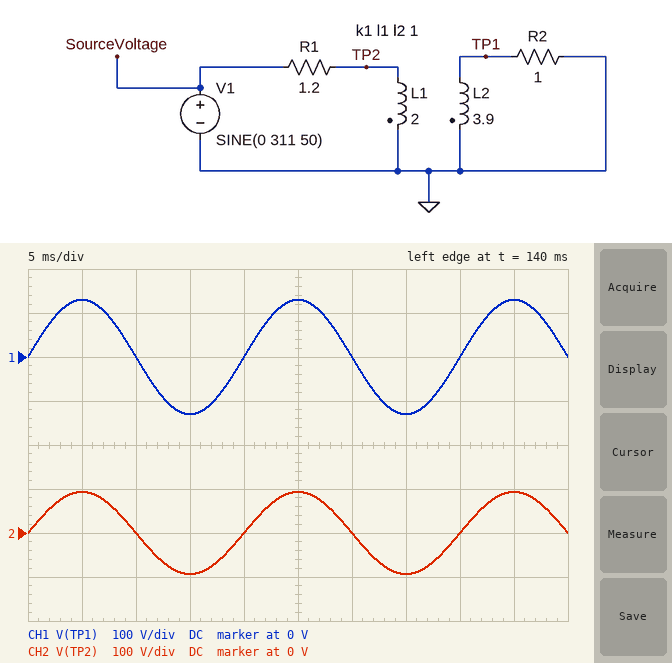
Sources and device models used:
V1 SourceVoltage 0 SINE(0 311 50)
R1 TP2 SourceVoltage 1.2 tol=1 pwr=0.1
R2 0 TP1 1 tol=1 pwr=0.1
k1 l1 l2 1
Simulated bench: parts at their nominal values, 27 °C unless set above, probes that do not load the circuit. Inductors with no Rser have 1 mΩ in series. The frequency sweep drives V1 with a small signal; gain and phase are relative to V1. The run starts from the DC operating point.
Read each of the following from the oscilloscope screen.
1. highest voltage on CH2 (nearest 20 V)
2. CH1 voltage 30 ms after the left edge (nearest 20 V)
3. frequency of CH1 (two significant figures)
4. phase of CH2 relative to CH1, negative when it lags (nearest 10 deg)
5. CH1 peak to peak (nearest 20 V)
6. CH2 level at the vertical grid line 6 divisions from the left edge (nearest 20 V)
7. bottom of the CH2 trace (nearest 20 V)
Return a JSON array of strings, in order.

["100 V", "0 V", "50 Hz", "0 deg", "260 V", "0 V", "-100 V"]
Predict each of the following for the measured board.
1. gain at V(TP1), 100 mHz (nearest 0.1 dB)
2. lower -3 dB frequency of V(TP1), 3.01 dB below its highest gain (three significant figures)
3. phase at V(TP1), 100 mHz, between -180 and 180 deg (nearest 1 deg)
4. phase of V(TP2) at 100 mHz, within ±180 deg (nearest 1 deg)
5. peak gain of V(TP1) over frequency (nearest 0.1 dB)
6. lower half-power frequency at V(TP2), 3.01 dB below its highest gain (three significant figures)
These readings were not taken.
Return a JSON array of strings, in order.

["-7.9 dB", "28.6 mHz", "16 deg", "16 deg", "-7.6 dB", "28.6 mHz"]
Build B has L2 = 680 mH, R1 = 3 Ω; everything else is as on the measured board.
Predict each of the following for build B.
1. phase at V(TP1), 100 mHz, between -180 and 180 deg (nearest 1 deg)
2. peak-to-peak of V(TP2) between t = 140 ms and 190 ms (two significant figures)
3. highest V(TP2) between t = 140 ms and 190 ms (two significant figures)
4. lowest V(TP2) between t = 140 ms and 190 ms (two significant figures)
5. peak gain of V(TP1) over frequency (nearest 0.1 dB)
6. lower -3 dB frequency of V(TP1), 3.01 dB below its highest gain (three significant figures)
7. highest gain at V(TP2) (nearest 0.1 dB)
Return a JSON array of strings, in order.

["50 deg", "310 V", "150 V", "-150 V", "-10.8 dB", "118 mHz", "-6.1 dB"]
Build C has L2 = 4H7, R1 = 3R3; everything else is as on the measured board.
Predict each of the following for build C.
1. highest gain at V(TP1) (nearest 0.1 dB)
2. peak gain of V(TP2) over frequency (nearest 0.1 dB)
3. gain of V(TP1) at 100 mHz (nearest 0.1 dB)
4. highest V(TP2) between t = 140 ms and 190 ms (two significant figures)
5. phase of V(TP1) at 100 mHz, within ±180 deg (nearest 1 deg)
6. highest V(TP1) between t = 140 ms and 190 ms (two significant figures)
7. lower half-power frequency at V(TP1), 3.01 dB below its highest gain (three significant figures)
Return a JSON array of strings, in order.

["-15.1 dB", "-18.8 dB", "-15.5 dB", "36 V", "17 deg", "54 V", "30.0 mHz"]
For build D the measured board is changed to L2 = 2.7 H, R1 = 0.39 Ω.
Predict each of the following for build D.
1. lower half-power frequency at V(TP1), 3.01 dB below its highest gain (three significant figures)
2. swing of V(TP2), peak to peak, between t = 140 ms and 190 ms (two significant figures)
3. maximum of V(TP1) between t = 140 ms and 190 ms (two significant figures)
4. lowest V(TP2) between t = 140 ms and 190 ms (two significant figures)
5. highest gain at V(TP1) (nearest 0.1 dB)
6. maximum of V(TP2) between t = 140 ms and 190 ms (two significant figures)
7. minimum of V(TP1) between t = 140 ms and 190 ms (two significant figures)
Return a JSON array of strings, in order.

["20.4 mHz", "410 V", "240 V", "-200 V", "-2.4 dB", "200 V", "-240 V"]
